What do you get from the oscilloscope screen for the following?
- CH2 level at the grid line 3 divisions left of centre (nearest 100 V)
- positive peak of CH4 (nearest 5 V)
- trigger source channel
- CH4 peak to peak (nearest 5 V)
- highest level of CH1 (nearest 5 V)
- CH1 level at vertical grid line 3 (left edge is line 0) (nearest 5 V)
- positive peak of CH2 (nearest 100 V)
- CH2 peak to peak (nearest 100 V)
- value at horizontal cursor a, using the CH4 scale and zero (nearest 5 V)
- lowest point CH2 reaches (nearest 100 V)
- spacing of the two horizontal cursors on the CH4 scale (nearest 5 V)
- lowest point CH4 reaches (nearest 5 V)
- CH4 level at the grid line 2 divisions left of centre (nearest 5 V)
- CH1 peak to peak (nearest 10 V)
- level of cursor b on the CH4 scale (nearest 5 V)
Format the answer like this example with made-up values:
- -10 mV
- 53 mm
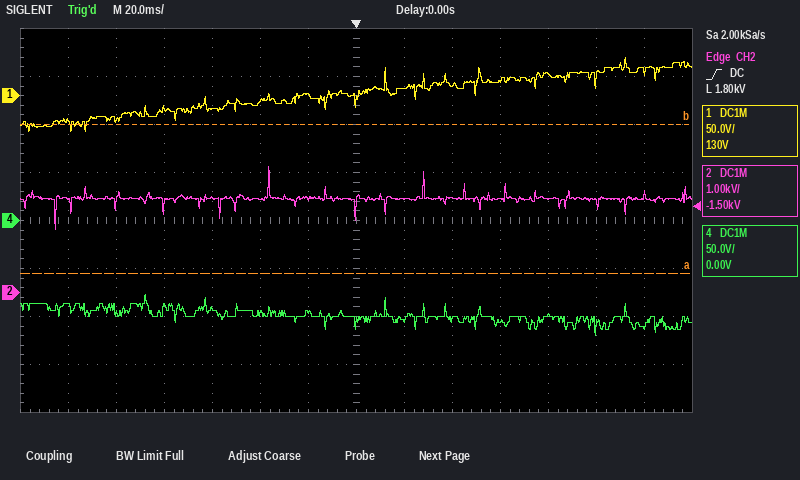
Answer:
- 2.0 kV
- -75 V
- CH2
- 45 V
- 40 V
- -15 V
- 2.6 kV
- 1.3 kV
- -55 V
- 1.3 kV
- 155 V
- -120 V
- -95 V
- 80 V
- 100 V
